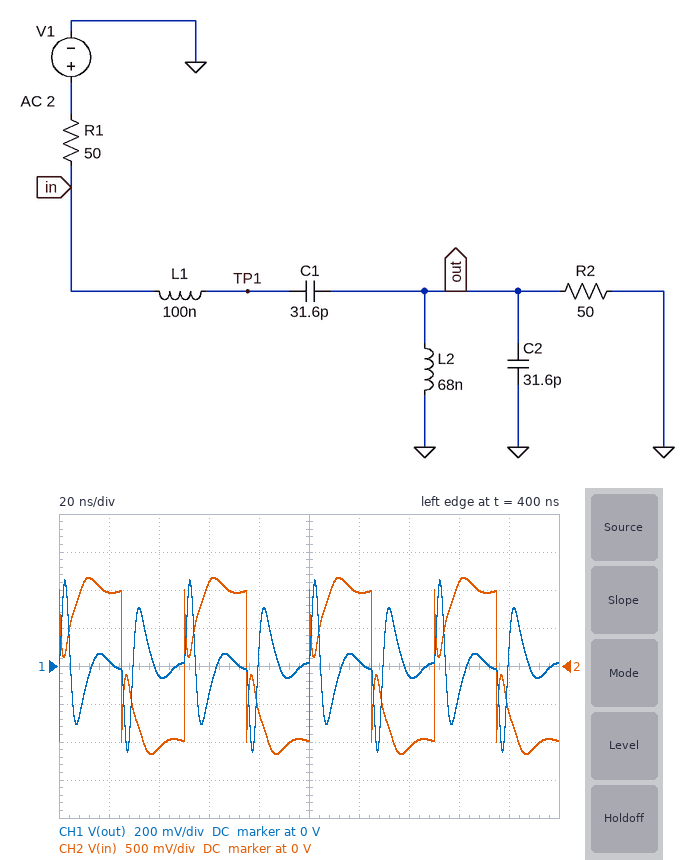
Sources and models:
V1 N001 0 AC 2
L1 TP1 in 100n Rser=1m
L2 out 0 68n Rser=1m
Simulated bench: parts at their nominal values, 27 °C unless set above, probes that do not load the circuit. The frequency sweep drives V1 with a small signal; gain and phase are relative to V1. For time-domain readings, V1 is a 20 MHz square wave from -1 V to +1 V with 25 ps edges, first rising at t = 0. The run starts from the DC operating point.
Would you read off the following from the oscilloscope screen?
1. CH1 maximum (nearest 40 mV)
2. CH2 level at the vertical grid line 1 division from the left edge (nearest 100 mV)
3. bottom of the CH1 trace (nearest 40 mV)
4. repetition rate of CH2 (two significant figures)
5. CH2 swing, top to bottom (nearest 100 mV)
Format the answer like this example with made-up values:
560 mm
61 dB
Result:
440 mV
1.0 V
-440 mV
20 MHz
2.3 V
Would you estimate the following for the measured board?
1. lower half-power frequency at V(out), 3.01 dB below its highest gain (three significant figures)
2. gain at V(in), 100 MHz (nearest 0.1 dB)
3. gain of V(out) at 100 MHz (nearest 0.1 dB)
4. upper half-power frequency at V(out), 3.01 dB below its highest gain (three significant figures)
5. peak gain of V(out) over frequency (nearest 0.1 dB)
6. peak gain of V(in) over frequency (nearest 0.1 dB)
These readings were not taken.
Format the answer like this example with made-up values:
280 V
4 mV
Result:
53.3 MHz
-5.6 dB
-6.2 dB
182 MHz
-6.2 dB
0 dB
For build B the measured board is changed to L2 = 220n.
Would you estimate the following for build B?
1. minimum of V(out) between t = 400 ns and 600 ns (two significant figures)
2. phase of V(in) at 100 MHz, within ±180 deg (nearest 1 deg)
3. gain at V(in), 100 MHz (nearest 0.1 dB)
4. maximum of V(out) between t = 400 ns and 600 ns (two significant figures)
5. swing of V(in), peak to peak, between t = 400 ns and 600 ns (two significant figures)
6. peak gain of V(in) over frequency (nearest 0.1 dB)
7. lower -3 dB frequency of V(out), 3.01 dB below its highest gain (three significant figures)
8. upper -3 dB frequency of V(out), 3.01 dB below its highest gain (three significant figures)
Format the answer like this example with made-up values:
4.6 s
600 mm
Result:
-530 mV
-9 deg
-7.3 dB
530 mV
2.1 V
0 dB
37.5 MHz
165 MHz
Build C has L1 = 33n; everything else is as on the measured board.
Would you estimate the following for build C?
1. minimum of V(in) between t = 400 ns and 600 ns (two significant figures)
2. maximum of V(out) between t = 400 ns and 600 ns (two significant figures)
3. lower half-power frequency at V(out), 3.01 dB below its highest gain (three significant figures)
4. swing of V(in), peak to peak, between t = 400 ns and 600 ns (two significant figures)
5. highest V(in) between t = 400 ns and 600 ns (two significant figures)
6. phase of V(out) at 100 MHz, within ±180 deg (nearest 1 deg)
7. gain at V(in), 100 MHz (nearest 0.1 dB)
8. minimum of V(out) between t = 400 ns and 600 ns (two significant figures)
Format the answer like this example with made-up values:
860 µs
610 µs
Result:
-1.1 V
540 mV
58.6 MHz
2.2 V
1.1 V
22 deg
-5.6 dB
-540 mV
